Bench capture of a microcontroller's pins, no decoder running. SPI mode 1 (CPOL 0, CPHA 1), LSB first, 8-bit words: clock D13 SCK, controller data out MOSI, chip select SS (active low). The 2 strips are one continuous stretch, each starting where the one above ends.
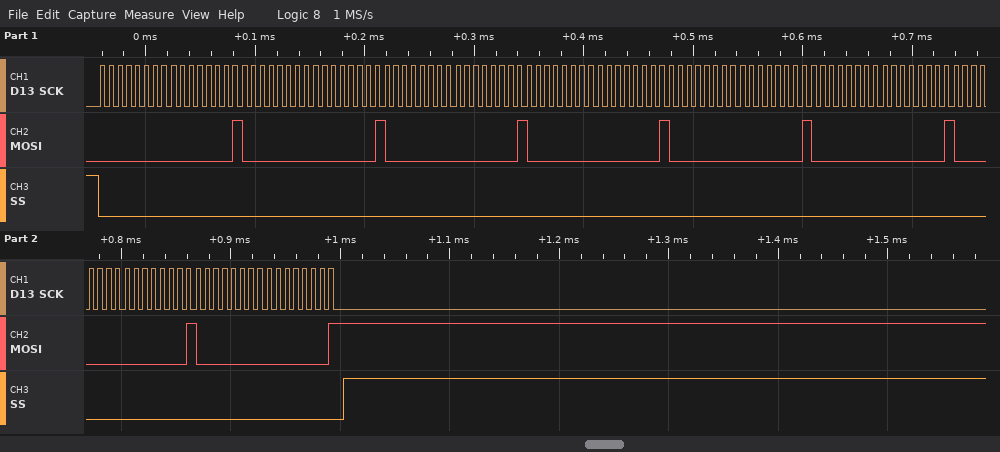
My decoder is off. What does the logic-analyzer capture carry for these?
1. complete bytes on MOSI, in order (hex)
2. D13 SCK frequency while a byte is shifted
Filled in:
00 80 00 80 00 80 00 80 00 80 00 80 00 80 00 80
125 kHz
